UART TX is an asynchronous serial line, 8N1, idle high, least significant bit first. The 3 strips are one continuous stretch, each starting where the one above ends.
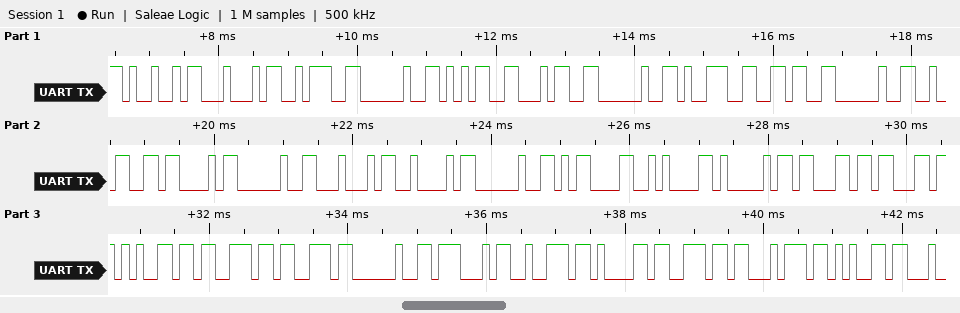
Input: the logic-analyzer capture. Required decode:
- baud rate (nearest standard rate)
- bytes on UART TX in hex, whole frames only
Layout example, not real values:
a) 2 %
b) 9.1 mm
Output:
a) 9600 baud
b) 49 44 3A 20 35 34 20 39 36 20 32 43 20 44 42 20 0D 0A 41 63 63 65 73 73 20 47 72 61 6E 74 65
